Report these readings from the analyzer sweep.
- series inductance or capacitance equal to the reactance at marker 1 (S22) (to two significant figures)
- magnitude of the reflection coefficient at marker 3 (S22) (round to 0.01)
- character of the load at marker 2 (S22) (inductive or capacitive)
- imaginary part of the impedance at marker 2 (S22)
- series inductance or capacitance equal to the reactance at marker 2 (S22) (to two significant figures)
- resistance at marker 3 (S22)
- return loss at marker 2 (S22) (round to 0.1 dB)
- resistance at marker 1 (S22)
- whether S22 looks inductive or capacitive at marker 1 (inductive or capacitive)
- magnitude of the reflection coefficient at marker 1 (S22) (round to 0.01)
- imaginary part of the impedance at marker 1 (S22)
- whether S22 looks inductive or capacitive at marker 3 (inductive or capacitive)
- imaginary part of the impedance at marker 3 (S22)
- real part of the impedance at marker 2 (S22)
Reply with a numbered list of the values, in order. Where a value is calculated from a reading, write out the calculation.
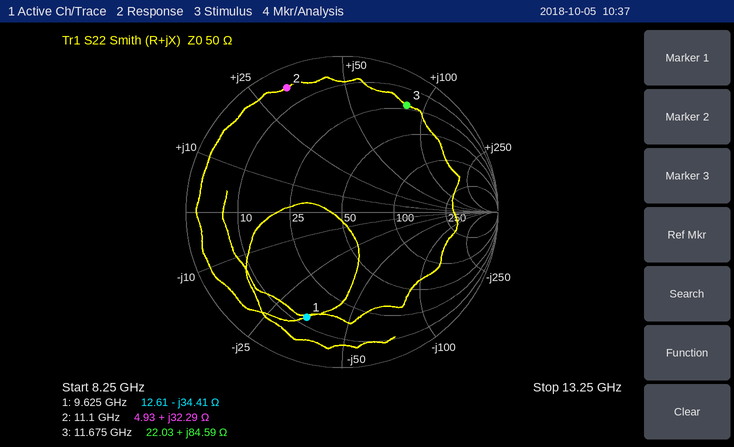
1. C = 1/(2π × 9.625 GHz × 34.41 Ω) ≈ 481 fF, so 480 fF to two significant figures
2. 0.80
3. inductive
4. +32.29 Ω
5. L = 32.29 Ω/(2π × 11.1 GHz) ≈ 463 pH, so 460 pH to two significant figures
6. 22.03 Ω
7. 1.2 dB
8. 12.61 Ω
9. capacitive
10. 0.71
11. -34.41 Ω
12. inductive
13. +84.59 Ω
14. 4.93 Ω
